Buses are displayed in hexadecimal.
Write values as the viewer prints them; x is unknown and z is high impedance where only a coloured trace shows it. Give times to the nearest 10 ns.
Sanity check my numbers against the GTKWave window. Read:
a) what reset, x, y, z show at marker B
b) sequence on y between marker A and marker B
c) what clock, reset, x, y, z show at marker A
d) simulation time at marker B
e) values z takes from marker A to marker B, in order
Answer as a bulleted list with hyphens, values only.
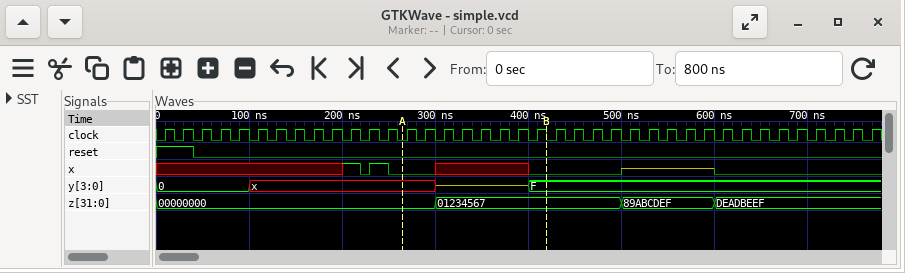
- reset=0, x=0, y=F, z=01234567
- x, z, F
- clock=0, reset=0, x=0, y=x, z=00000000
- 420 ns
- 00000000, 01234567
